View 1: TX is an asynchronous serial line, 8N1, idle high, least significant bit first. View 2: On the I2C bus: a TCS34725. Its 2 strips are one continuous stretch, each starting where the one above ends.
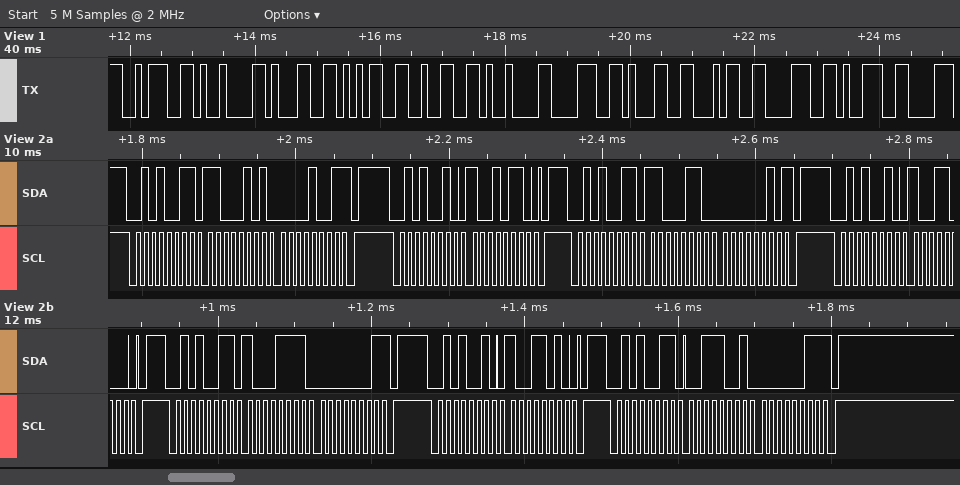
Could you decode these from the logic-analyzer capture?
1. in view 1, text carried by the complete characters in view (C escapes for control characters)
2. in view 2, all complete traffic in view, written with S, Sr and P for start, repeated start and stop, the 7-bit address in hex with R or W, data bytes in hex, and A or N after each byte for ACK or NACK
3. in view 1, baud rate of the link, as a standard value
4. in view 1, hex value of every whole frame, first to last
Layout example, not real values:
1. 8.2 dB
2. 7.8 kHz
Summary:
1. ":\t152\t81489"
2. S 29R A C5 A 09 N P S 29W A 96 A P S 29R A C6 A 02 N P S 29W A 98 A P S 29R A 8F A 01 N P S 29W A 9A A P S 29R A 39 A 03 N P
3. 9600 baud
4. 0x3A 0x09 0x31 0x35 0x32 0x09 0x38 0x31 0x34 0x38 0x39
